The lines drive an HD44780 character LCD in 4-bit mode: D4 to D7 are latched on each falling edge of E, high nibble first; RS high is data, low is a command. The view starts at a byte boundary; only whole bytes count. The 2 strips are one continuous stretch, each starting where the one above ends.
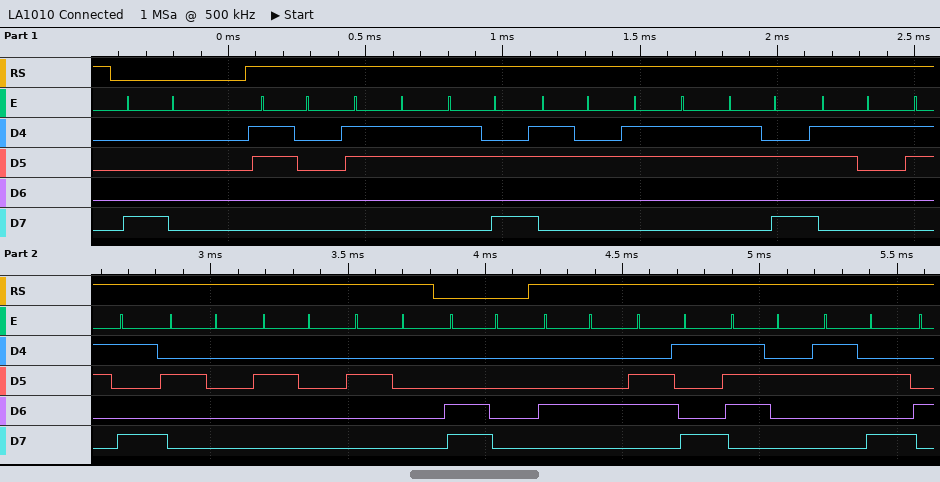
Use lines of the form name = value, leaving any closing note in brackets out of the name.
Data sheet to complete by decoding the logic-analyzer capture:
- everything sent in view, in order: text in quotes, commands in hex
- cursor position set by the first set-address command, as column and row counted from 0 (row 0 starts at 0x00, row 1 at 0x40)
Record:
everything sent in view, in order: text in quotes, commands in hex = 0x80 "03:23:19   " 0xC0 "Dir:"
cursor position set by the first set-address command, as column and row counted from 0 = column 0, row 0
